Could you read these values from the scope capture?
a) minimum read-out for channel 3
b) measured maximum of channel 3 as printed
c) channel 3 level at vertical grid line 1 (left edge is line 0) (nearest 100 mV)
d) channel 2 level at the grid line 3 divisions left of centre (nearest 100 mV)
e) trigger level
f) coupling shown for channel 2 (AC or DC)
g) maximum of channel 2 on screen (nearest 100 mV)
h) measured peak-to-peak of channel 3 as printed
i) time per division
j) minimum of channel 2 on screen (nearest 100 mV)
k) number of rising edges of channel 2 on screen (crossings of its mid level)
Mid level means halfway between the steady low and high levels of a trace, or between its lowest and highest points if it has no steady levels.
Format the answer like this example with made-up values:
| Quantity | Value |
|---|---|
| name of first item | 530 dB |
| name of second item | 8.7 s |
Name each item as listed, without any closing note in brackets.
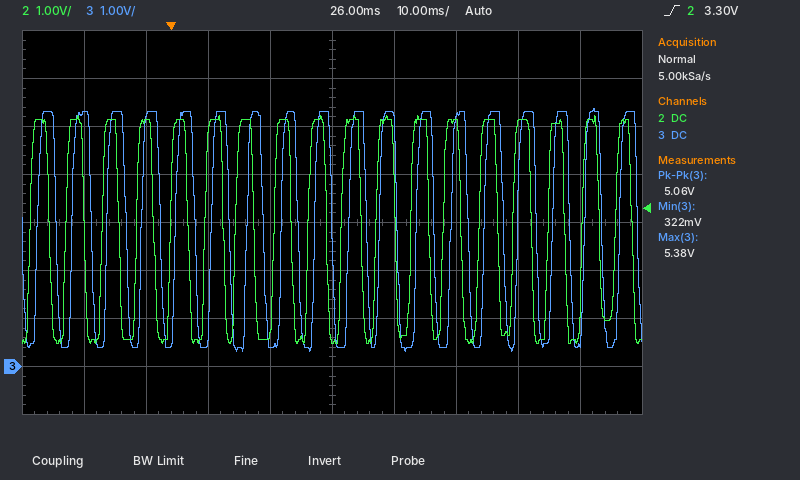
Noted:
| Quantity | Value |
|---|---|
| minimum read-out for channel 3 | 322 mV |
| measured maximum of channel 3 as printed | 5.38 V |
| channel 3 level at vertical grid line 1 (left edge is line 0) | 5.3 V |
| channel 2 level at the grid line 3 divisions left of centre | 5.1 V |
| trigger level | 3.30 V |
| coupling shown for channel 2 | DC |
| maximum of channel 2 on screen | 5.2 V |
| measured peak-to-peak of channel 3 as printed | 5.06 V |
| time per division | 10 ms |
| minimum of channel 2 on screen | 500 mV |
| number of rising edges of channel 2 on screen | 18 |
